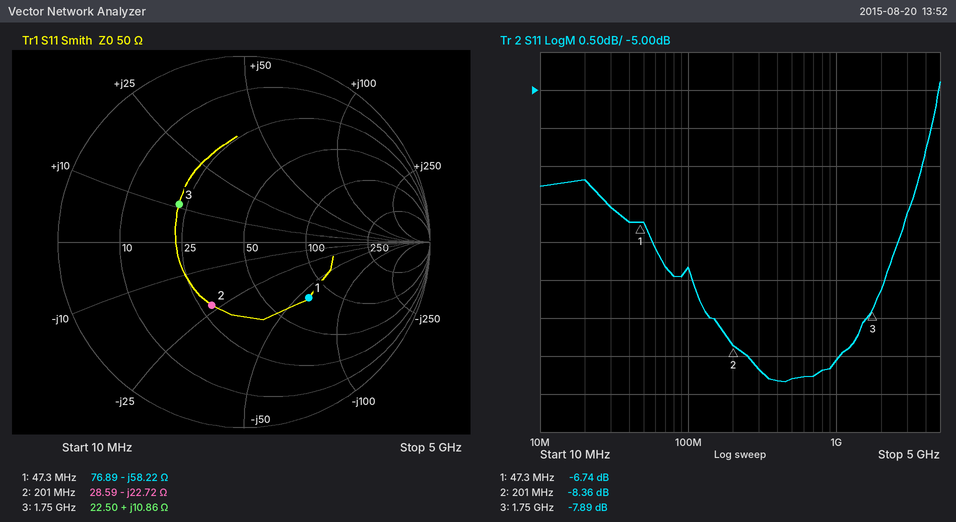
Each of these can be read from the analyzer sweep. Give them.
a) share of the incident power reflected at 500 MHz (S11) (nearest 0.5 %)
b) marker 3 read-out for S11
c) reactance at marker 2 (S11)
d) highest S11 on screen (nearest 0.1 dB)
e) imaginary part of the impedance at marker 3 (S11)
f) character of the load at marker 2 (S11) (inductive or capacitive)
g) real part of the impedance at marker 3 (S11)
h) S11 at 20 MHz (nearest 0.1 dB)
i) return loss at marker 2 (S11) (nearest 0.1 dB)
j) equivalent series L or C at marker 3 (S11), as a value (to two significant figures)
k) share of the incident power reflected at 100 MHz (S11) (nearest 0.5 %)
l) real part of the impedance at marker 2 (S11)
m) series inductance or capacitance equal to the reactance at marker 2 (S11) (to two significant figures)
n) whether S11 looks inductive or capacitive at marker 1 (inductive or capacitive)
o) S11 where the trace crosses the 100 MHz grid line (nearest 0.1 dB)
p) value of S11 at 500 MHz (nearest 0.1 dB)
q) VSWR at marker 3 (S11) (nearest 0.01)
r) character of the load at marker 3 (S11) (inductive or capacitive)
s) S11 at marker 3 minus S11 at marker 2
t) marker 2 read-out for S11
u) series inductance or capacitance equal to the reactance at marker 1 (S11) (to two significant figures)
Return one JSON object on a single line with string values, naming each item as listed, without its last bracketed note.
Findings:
{"share of the incident power reflected at 500 MHz (S11)": "13.0 %", "marker 3 read-out for S11": "-7.89 dB", "reactance at marker 2": "-22.72 Ω", "highest S11 on screen": "-4.9 dB", "imaginary part of the impedance at marker 3": "+10.86 Ω", "character of the load at marker 2 (S11)": "capacitive", "real part of the impedance at marker 3": "22.50 Ω", "S11 at 20 MHz": "-6.2 dB", "return loss at marker 2 (S11)": "8.4 dB", "equivalent series L or C at marker 3 (S11), as a value": "990 pH", "share of the incident power reflected at 100 MHz (S11)": "18.5 %", "real part of the impedance at marker 2": "28.59 Ω", "series inductance or capacitance equal to the reactance at marker 2 (S11)": "35 pF", "whether S11 looks inductive or capacitive at marker 1": "capacitive", "S11 where the trace crosses the 100 MHz grid line": "-7.3 dB", "value of S11 at 500 MHz": "-8.8 dB", "VSWR at marker 3 (S11)": "2.35", "character of the load at marker 3 (S11)": "inductive", "S11 at marker 3 minus S11 at marker 2": "0.47 dB", "marker 2 read-out for S11": "-8.36 dB", "series inductance or capacitance equal to the reactance at marker 1 (S11)": "58 pF"}
